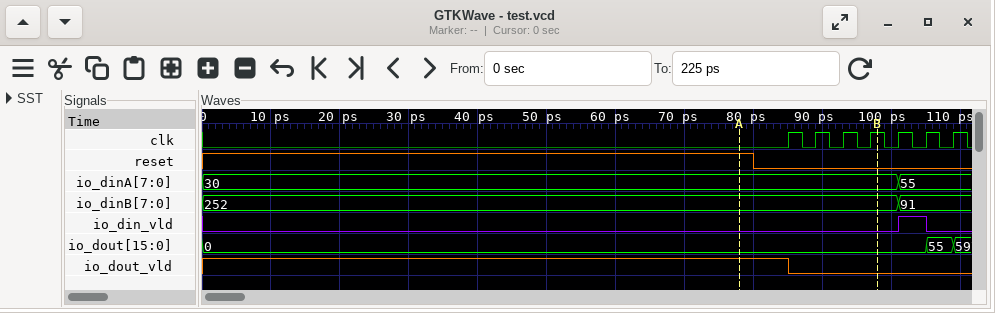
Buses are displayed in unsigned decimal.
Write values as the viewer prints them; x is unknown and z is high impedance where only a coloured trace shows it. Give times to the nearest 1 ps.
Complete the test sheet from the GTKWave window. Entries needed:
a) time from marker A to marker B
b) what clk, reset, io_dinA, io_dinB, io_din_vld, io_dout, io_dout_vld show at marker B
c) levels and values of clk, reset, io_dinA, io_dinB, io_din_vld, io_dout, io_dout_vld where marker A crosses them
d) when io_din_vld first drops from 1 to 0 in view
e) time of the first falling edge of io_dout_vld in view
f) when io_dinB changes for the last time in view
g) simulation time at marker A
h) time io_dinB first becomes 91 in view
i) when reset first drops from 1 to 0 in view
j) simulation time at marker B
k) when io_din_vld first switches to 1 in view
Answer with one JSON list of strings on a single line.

["20 ps", "clk=1, reset=0, io_dinA=30, io_dinB=252, io_din_vld=0, io_dout=0, io_dout_vld=0", "clk=0, reset=1, io_dinA=30, io_dinB=252, io_din_vld=0, io_dout=0, io_dout_vld=1", "105 ps", "85 ps", "101 ps", "78 ps", "101 ps", "80 ps", "98 ps", "101 ps"]
